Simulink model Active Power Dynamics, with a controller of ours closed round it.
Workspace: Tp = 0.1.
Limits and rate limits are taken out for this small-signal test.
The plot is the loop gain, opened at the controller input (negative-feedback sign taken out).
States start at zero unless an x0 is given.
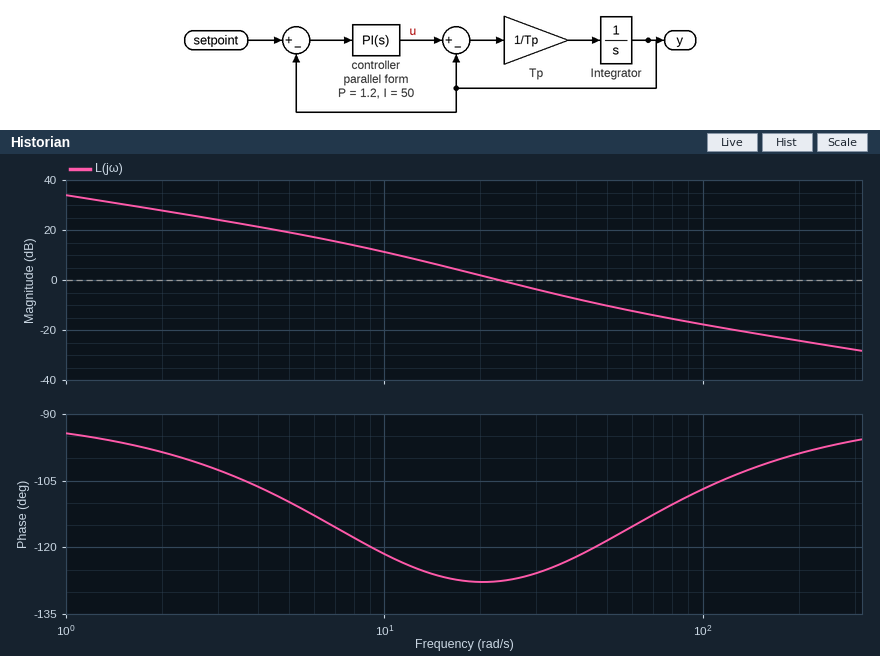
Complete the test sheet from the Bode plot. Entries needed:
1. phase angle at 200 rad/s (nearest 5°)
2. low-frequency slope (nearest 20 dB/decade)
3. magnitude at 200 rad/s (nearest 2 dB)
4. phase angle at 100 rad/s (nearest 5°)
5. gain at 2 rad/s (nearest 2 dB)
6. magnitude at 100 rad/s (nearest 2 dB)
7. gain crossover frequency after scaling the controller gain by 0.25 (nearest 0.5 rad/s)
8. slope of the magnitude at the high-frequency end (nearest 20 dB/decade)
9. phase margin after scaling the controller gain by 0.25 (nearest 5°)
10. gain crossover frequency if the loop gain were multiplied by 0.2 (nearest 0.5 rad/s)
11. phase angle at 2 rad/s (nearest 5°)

-100°
-20 dB/decade
-24 dB
-105°
28 dB
-18 dB
9.5 rad/s
-20 dB/decade
60°
8.0 rad/s
-100°
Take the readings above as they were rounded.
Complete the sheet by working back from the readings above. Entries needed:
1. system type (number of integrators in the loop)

1
